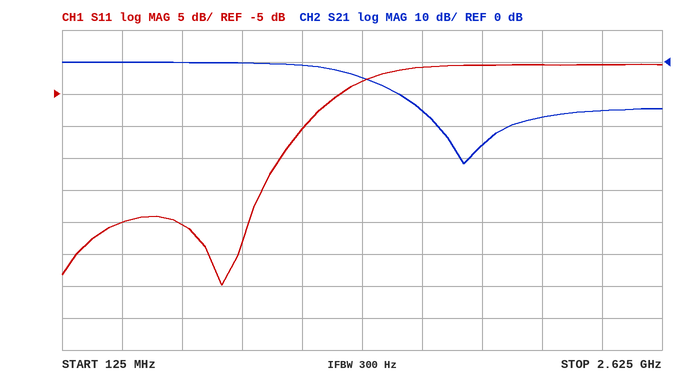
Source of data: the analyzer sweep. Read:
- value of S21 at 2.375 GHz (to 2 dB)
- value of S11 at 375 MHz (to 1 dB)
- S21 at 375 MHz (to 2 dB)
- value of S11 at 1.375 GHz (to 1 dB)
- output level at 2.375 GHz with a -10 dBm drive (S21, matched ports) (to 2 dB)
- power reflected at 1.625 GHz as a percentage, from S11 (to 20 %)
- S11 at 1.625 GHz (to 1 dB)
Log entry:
-16 dB
-25 dB
0 dB
-3 dB
-26 dBm
80 %
-1 dB
